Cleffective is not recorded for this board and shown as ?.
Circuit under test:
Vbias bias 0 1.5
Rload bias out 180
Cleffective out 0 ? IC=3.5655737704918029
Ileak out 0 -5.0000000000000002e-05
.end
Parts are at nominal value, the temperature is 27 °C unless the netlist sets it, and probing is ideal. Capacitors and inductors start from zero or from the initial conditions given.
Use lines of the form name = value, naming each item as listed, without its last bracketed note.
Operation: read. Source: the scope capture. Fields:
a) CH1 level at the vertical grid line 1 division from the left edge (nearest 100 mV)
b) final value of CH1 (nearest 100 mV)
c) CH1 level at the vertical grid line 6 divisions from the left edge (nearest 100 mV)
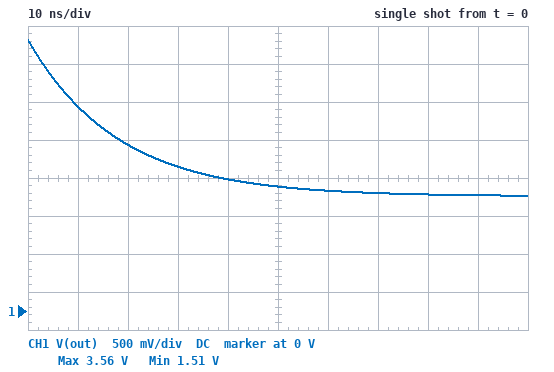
CH1 level at the vertical grid line 1 division from the left edge = 2.7 V
final value of CH1 = 1.5 V
CH1 level at the vertical grid line 6 divisions from the left edge = 1.6 V
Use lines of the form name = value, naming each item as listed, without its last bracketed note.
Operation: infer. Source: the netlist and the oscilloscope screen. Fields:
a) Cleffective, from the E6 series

Cleffective, from the E6 series = 100 pF
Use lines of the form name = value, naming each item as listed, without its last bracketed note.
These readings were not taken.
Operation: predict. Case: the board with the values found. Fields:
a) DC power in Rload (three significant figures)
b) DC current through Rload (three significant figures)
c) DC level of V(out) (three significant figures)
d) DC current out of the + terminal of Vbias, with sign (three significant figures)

DC power in Rload = 450 nW
DC current through Rload = 50.0 µA
DC level of V(out) = 1.51 V
DC current out of the + terminal of Vbias, with sign = -50.0 µA
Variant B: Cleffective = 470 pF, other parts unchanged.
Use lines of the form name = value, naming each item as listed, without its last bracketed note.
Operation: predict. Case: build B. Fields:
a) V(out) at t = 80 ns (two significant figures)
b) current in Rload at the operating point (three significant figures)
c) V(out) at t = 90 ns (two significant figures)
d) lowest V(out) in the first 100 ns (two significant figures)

V(out) at t = 80 ns = 2.3 V
current in Rload at the operating point = 50.0 µA
V(out) at t = 90 ns = 2.2 V
lowest V(out) in the first 100 ns = 2.1 V
